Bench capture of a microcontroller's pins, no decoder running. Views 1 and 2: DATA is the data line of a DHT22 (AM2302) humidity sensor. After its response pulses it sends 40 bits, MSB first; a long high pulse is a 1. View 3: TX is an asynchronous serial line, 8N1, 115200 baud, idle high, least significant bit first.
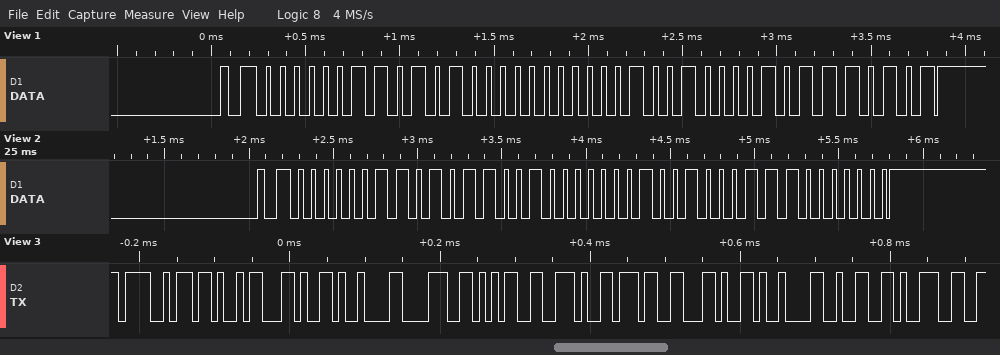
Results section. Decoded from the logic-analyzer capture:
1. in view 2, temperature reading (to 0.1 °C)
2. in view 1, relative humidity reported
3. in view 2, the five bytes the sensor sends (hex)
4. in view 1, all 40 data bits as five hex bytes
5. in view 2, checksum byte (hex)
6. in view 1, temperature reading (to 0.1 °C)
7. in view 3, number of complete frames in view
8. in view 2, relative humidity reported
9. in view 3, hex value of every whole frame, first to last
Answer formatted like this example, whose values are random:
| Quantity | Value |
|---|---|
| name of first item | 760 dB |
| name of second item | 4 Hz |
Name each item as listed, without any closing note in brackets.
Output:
| Quantity | Value |
|---|---|
| in view 2, temperature reading | 29.1 °C |
| in view 1, relative humidity reported | 84.8 % |
| in view 2, the five bytes the sensor sends | 03 59 01 23 80 |
| in view 1, all 40 data bits as five hex bytes | 03 50 01 21 75 |
| in view 2, checksum byte | 0x80 |
| in view 1, temperature reading | 28.9 °C |
| in view 3, number of complete frames in view | 12 |
| in view 2, relative humidity reported | 85.7 % |
| in view 3, hex value of every whole frame, first to last | 4F 4B 2C 09 38 35 2E 37 2C 09 32 39 |
